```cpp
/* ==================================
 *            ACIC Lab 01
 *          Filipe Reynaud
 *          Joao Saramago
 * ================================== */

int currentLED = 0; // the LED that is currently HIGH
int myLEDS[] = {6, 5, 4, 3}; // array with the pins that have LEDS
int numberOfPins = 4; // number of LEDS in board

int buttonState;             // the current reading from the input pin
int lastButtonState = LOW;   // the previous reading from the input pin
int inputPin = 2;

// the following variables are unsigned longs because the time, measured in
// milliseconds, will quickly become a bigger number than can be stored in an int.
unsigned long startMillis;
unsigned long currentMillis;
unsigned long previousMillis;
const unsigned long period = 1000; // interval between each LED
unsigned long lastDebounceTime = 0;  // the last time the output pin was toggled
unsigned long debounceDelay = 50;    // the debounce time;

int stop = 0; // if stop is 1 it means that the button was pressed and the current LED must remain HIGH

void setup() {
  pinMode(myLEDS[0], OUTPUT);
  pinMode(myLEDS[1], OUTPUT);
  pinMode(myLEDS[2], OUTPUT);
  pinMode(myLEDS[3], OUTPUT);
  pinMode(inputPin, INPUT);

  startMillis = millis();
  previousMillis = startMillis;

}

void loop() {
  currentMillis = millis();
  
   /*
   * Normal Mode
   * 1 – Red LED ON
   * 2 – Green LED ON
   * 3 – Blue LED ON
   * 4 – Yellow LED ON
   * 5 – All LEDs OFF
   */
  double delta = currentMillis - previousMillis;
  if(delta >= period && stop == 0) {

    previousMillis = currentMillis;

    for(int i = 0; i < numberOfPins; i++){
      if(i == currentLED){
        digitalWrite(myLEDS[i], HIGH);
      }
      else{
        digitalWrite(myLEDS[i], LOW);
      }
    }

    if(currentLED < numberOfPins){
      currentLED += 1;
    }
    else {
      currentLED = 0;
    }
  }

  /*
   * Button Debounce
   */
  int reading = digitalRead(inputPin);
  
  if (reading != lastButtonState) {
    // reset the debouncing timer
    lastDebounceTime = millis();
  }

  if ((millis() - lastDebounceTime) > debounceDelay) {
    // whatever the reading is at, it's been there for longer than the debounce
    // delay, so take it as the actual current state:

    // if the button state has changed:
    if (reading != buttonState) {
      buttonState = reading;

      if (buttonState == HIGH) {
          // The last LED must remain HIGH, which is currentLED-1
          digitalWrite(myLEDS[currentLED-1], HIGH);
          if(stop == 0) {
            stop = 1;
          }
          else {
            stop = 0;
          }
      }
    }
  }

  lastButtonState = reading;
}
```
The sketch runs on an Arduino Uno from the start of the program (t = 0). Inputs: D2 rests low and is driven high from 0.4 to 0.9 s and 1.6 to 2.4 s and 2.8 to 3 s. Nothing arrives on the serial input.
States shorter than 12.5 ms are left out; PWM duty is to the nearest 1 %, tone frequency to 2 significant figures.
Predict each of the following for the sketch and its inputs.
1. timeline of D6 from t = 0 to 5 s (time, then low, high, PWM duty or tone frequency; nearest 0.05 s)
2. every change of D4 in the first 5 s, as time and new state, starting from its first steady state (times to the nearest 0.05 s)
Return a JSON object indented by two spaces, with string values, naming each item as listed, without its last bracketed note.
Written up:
{
  "timeline of D6 from t = 0 to 5 s": "0 s low; 1.65 s high; 2.65 s low",
  "every change of D4 in the first 5 s, as time and new state, starting from its first steady state": "0 s low; 0.45 s high; 1.65 s low"
}
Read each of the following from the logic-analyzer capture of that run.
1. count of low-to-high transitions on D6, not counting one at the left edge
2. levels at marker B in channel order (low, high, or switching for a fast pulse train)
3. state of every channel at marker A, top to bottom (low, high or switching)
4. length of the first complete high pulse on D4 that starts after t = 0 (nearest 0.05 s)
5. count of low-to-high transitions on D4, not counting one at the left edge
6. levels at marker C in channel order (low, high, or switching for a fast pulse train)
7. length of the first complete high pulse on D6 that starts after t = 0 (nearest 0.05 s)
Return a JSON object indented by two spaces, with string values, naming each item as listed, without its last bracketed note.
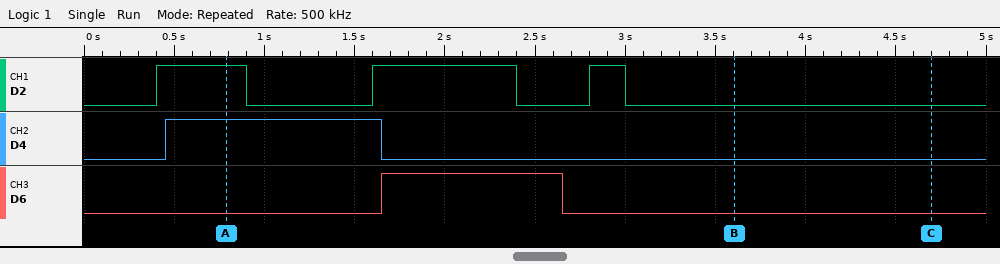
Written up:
{
  "count of low-to-high transitions on D6, not counting one at the left edge": "1",
  "levels at marker B in channel order": "D2 low, D4 low, D6 low",
  "state of every channel at marker A, top to bottom": "D2 high, D4 high, D6 low",
  "length of the first complete high pulse on D4 that starts after t = 0": "1.20 s",
  "count of low-to-high transitions on D4, not counting one at the left edge": "1",
  "levels at marker C in channel order": "D2 low, D4 low, D6 low",
  "length of the first complete high pulse on D6 that starts after t = 0": "1.00 s"
}
